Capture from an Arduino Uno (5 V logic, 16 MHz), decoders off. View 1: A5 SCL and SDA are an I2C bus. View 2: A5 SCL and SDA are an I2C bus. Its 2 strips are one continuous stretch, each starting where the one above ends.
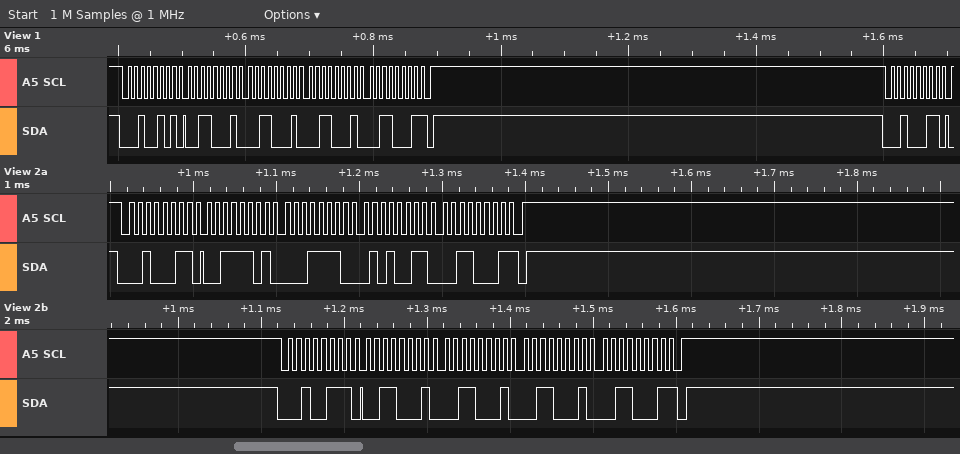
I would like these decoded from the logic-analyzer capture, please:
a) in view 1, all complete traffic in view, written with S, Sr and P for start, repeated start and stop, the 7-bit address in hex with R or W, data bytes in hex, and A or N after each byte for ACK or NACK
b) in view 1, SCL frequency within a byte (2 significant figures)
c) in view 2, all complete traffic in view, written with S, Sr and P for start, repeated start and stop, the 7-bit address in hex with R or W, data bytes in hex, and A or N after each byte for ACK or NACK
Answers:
S 12R A 31 A 31 A 31 A 31 N P S 11R A
100 kHz
S 11R A 3D A 1E A 53 A 31 N P S 13R A 31 A 31 A 31 A 31 N P
